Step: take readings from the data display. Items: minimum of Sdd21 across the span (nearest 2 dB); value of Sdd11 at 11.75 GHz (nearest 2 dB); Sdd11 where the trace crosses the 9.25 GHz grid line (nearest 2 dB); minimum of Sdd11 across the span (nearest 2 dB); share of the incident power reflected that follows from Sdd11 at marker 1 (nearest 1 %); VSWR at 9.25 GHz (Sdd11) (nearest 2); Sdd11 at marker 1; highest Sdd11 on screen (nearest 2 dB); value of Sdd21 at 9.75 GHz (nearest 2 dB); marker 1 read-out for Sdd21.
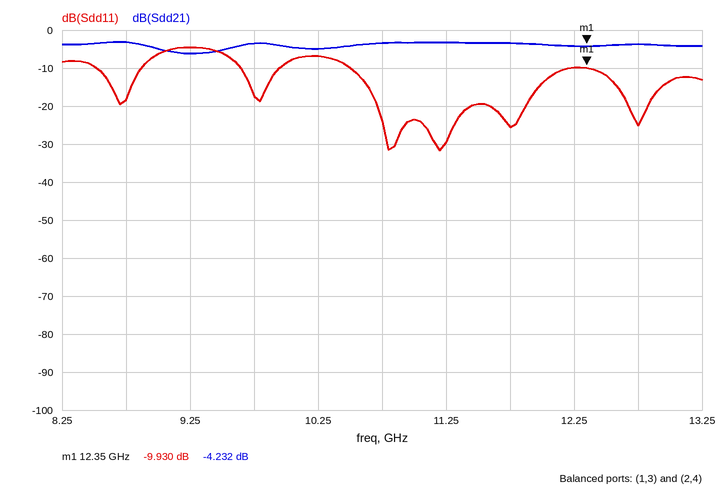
-6 dB
-26 dB
-4 dB
-32 dB
10 %
4
-9.930 dB
-4 dB
-4 dB
-4.232 dB
